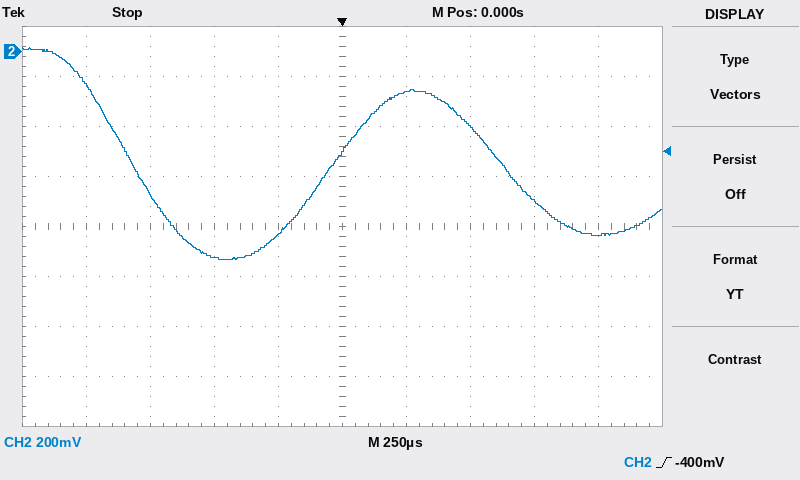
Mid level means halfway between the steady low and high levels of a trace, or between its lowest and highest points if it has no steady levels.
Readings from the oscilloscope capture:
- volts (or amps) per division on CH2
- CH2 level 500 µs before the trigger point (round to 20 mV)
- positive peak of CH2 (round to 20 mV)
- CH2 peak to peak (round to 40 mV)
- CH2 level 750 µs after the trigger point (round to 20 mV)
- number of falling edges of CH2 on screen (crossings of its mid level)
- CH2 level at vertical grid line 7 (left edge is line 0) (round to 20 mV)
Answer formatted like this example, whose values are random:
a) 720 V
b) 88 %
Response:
a) 200 mV
b) -820 mV
c) 20 mV
d) 840 mV
e) -600 mV
f) 2
g) -300 mV
